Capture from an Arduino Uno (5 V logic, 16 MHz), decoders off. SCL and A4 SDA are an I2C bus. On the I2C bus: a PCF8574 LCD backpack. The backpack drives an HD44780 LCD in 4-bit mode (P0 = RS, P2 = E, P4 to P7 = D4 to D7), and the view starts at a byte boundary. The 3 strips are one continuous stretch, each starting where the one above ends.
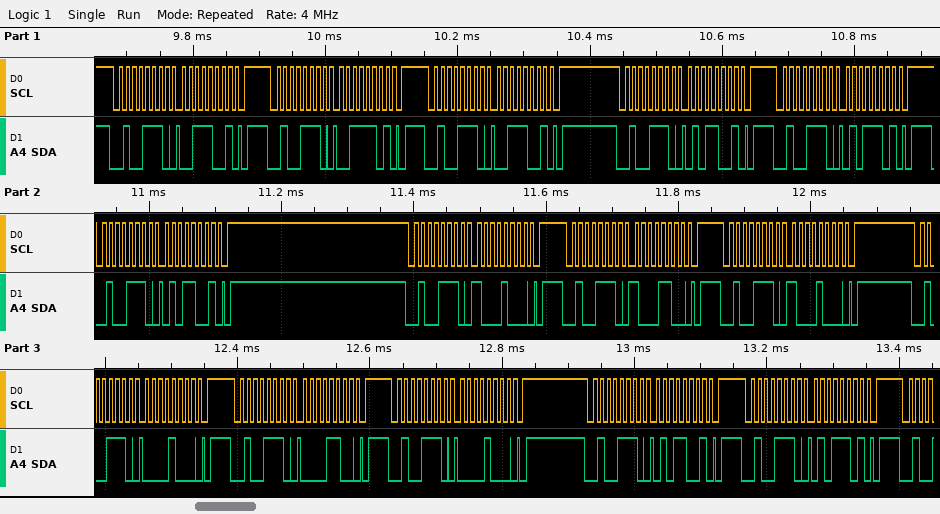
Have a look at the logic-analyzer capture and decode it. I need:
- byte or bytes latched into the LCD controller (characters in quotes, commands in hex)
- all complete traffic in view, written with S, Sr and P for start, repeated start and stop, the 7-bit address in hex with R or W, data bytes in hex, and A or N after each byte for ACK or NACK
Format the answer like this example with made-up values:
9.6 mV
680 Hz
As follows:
'5' 0x80
S 27W A 39 A P S 27W A 3D A P S 27W A 39 A P S 27W A 59 A P S 27W A 5D A P S 27W A 59 A P S 27W A 88 A P S 27W A 8C A P S 27W A 88 A P S 27W A 08 A P S 27W A 0C A P S 27W A 08 A P S 27W A 59 A P S 27W A 5D A P
